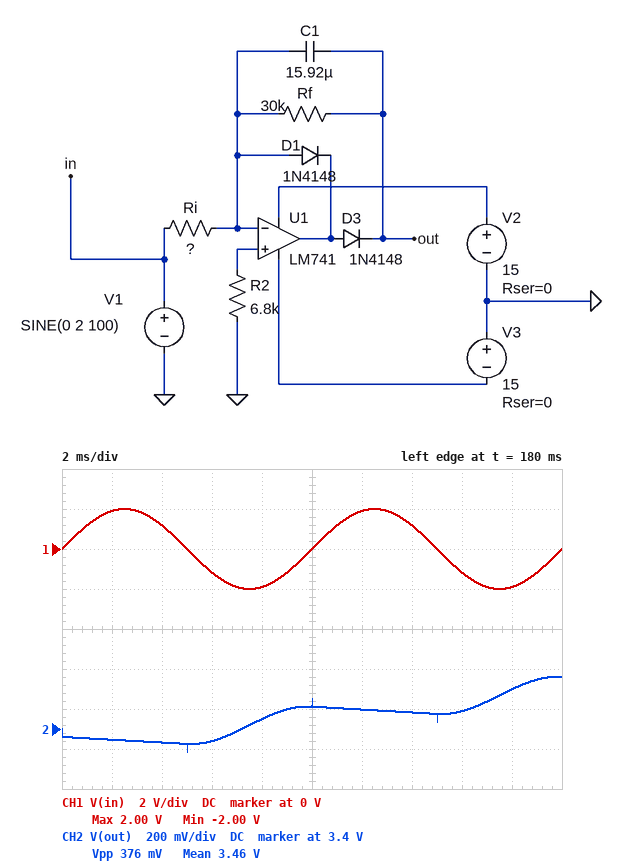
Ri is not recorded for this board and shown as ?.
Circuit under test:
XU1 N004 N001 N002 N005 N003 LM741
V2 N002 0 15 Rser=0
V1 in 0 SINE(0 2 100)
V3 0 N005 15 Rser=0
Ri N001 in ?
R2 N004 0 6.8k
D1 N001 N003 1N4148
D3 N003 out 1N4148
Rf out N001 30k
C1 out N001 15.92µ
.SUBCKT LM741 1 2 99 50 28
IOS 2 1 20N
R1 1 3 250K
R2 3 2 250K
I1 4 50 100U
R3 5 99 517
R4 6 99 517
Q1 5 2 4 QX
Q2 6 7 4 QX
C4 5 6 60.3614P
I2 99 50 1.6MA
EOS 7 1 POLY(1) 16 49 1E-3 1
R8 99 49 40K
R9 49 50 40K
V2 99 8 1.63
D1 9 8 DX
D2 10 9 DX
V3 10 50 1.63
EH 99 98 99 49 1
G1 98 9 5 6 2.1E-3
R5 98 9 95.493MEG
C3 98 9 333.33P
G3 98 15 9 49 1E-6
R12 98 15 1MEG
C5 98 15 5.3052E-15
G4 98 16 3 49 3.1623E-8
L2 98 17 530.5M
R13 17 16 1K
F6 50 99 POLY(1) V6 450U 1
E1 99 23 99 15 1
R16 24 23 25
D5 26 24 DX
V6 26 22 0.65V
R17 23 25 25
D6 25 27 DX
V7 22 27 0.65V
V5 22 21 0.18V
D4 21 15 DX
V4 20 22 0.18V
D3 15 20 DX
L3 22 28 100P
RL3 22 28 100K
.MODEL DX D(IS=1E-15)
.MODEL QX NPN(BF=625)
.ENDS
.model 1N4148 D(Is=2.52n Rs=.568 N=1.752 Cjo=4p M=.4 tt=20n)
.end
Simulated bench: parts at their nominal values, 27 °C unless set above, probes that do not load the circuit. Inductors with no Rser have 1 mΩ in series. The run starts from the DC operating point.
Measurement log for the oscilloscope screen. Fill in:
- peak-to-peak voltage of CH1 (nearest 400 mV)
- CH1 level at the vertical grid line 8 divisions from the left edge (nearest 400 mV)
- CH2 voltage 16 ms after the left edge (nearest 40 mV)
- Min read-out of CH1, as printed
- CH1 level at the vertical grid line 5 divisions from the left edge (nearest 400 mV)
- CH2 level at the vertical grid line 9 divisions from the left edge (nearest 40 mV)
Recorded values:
4.0 V
-1.2 V
3.48 V
-2.00 V
0 V
3.60 V
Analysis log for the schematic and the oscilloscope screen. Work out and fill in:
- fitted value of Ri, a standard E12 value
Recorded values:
1.8 kΩ
